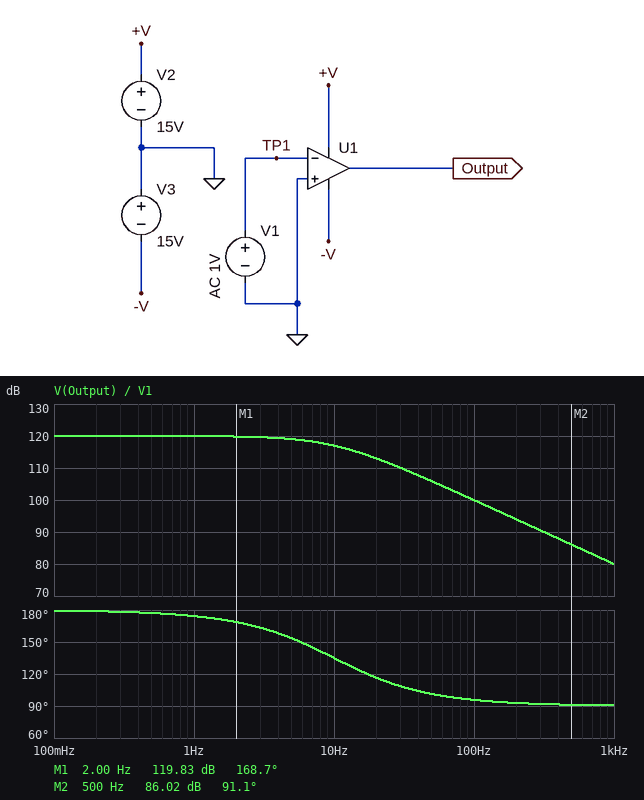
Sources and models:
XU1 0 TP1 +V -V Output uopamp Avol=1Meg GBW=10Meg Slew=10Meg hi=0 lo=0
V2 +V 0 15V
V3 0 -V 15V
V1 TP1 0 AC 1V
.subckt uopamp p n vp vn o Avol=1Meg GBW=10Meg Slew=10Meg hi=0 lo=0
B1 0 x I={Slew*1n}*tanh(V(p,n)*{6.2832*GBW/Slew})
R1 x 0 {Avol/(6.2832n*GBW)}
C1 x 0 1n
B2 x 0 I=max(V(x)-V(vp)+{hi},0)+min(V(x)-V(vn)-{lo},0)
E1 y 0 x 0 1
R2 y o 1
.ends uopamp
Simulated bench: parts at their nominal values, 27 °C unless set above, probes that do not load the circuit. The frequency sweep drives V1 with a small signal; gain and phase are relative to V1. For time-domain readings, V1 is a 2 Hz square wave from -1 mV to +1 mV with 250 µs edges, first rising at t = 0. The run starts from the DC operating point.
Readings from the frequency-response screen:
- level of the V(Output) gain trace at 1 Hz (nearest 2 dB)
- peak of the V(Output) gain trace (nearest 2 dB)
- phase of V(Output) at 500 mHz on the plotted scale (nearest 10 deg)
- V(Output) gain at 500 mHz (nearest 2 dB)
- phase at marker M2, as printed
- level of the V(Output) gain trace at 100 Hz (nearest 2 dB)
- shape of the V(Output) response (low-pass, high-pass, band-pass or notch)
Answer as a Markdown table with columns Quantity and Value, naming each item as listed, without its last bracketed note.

| Quantity | Value |
|---|---|
| level of the V(Output) gain trace at 1 Hz | 120 dB |
| peak of the V(Output) gain trace | 120 dB |
| phase of V(Output) at 500 mHz on the plotted scale | 180 deg |
| V(Output) gain at 500 mHz | 120 dB |
| phase at marker M2, as printed | 91.1 deg |
| level of the V(Output) gain trace at 100 Hz | 100 dB |
| shape of the V(Output) response | low-pass |
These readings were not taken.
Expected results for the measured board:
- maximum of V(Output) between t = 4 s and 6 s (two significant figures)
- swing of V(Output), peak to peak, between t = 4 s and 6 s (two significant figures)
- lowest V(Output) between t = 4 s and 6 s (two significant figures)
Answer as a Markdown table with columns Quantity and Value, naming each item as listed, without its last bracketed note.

| Quantity | Value |
|---|---|
| maximum of V(Output) between t = 4 s and 6 s | 15 V |
| swing of V(Output), peak to peak, between t = 4 s and 6 s | 30 V |
| lowest V(Output) between t = 4 s and 6 s | -15 V |
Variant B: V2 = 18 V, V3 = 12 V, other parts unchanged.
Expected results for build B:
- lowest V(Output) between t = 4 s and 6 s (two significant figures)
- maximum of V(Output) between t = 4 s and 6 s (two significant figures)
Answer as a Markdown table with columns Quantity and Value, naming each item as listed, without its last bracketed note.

| Quantity | Value |
|---|---|
| lowest V(Output) between t = 4 s and 6 s | -12 V |
| maximum of V(Output) between t = 4 s and 6 s | 18 V |
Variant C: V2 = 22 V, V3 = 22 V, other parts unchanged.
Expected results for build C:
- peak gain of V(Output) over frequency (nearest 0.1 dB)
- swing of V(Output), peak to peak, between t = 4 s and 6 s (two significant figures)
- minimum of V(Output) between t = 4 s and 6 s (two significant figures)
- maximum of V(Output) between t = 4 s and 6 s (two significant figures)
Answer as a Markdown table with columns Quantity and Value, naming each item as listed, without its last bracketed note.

| Quantity | Value |
|---|---|
| peak gain of V(Output) over frequency | 120.0 dB |
| swing of V(Output), peak to peak, between t = 4 s and 6 s | 44 V |
| minimum of V(Output) between t = 4 s and 6 s | -22 V |
| maximum of V(Output) between t = 4 s and 6 s | 22 V |
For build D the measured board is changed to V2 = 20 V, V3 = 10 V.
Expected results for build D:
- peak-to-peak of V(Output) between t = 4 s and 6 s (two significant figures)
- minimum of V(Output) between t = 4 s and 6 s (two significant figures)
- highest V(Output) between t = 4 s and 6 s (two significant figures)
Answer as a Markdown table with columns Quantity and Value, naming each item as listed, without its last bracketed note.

| Quantity | Value |
|---|---|
| peak-to-peak of V(Output) between t = 4 s and 6 s | 30 V |
| minimum of V(Output) between t = 4 s and 6 s | -10 V |
| highest V(Output) between t = 4 s and 6 s | 20 V |
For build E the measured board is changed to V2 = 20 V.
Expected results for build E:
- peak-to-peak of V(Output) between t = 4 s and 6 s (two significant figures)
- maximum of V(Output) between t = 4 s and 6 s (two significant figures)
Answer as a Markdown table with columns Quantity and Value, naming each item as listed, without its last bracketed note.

| Quantity | Value |
|---|---|
| peak-to-peak of V(Output) between t = 4 s and 6 s | 35 V |
| maximum of V(Output) between t = 4 s and 6 s | 20 V |
